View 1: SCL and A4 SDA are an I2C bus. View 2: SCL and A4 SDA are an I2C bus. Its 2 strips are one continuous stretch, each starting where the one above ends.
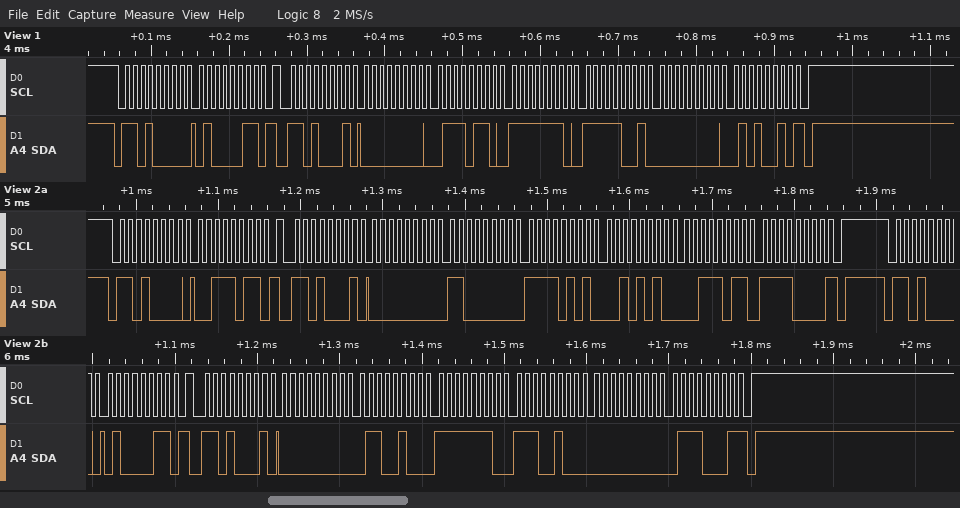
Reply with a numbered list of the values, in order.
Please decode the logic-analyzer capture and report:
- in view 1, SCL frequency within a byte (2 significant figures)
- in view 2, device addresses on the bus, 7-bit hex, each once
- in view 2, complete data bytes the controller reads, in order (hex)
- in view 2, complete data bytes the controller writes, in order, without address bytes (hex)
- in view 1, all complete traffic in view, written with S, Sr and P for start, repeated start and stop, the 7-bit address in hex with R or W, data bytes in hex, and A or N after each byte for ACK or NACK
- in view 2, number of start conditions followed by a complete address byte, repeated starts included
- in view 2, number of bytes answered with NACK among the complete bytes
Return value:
1. 100 kHz
2. 0x68
3. 00 C0 F5 2A 3B F0 00 64 FE E4 00 71
4. 3B 43
5. S 68W A 43 A Sr 68R A 00 A 76 A FE A F9 A 00 A 52 N P
6. 4
7. 2
